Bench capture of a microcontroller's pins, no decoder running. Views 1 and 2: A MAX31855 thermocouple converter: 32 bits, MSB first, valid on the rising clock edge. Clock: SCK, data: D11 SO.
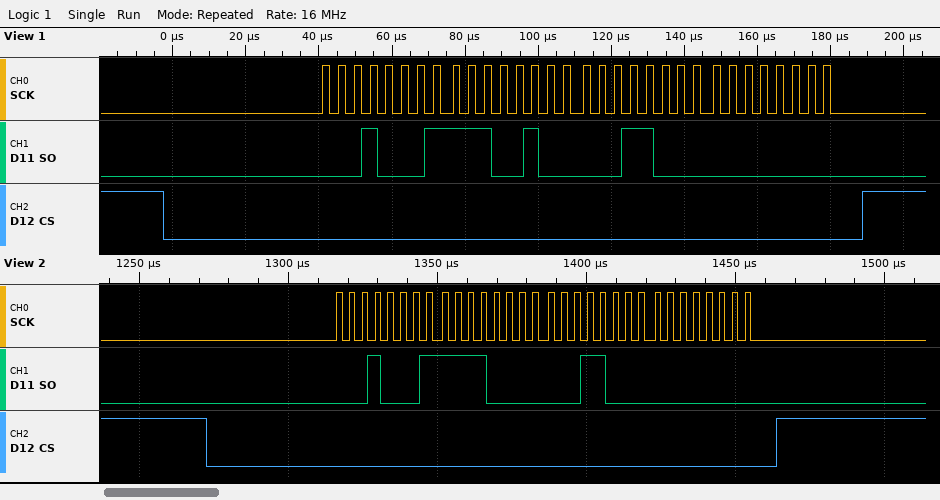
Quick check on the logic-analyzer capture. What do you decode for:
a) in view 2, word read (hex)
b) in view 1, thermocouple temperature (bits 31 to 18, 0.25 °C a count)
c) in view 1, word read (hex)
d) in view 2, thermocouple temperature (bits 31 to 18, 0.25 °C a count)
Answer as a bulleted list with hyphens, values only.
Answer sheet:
- 0x11F01800
- 286.25 °C
- 0x11E41800
- 287.00 °C
